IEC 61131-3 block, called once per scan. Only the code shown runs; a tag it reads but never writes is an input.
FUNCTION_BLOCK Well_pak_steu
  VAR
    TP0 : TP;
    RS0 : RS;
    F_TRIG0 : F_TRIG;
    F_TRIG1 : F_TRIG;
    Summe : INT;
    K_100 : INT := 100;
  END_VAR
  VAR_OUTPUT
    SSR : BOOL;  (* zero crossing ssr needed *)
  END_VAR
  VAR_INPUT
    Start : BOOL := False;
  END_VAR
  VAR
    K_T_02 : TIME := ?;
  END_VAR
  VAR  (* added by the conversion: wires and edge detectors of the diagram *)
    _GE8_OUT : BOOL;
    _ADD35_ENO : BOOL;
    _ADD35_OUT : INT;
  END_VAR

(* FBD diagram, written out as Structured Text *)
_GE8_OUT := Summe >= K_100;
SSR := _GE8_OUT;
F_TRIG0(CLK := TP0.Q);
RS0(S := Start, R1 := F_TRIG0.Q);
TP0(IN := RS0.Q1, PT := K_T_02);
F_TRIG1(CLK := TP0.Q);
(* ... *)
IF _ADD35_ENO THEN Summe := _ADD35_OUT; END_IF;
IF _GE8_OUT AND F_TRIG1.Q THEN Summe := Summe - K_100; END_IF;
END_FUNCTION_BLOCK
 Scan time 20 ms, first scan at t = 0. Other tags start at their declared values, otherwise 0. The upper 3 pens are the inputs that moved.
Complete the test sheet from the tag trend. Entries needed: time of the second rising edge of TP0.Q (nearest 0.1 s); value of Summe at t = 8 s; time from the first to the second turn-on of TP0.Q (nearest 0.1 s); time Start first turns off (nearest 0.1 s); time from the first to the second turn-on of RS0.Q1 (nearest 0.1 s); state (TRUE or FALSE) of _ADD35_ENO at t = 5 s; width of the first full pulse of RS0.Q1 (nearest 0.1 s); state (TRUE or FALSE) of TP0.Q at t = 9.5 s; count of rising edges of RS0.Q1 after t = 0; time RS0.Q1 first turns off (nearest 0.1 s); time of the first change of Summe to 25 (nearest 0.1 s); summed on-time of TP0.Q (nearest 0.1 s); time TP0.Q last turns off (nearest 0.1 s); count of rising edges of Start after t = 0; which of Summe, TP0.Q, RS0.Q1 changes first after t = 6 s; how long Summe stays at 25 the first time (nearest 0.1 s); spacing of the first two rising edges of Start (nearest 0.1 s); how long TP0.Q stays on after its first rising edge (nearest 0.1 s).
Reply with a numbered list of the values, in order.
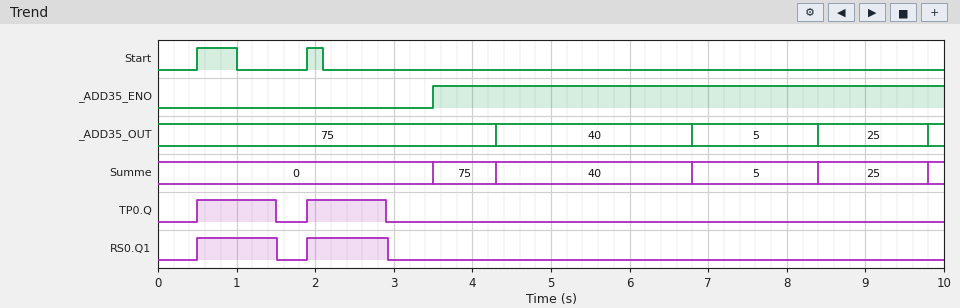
1. 1.9 s
2. 5
3. 1.4 s
4. 1.0 s
5. 1.4 s
6. TRUE
7. 1.0 s
8. FALSE
9. 2
10. 1.5 s
11. 8.4 s
12. 2.0 s
13. 2.9 s
14. 2
15. Summe
16. 1.4 s
17. 1.4 s
18. 1.0 s
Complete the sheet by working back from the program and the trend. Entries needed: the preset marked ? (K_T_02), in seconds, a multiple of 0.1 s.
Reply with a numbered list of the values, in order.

1. 1.0 s
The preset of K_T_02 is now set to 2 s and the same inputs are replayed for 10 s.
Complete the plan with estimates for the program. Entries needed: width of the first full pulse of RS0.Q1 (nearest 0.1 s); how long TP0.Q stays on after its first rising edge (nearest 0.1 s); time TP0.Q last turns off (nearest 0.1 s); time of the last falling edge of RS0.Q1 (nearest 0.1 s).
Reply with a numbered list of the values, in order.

1. 2.0 s
2. 2.0 s
3. 2.5 s
4. 2.5 s
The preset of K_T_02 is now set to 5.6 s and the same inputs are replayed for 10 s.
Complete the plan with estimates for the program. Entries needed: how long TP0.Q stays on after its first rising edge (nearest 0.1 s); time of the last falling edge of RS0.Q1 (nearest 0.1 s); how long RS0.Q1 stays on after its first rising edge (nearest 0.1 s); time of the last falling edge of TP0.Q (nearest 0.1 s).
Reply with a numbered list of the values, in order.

1. 5.6 s
2. 6.1 s
3. 5.6 s
4. 6.1 s
